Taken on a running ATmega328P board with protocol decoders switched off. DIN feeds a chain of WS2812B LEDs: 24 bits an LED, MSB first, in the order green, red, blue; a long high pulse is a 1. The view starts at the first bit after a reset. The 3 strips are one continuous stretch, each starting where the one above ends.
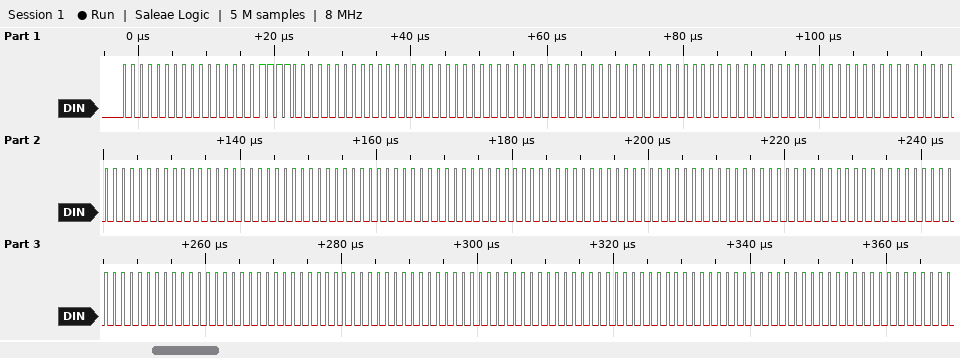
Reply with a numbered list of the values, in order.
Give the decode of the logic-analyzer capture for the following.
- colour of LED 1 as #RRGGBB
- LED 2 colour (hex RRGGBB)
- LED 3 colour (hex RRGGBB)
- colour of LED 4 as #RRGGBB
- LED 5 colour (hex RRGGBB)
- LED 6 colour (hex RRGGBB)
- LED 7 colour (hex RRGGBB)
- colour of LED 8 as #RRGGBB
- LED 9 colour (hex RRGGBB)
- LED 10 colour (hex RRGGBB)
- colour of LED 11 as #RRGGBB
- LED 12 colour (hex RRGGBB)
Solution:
1. #0000F0
2. #000000
3. #000000
4. #000000
5. #000000
6. #000000
7. #000000
8. #000000
9. #000000
10. #000000
11. #000000
12. #000000
